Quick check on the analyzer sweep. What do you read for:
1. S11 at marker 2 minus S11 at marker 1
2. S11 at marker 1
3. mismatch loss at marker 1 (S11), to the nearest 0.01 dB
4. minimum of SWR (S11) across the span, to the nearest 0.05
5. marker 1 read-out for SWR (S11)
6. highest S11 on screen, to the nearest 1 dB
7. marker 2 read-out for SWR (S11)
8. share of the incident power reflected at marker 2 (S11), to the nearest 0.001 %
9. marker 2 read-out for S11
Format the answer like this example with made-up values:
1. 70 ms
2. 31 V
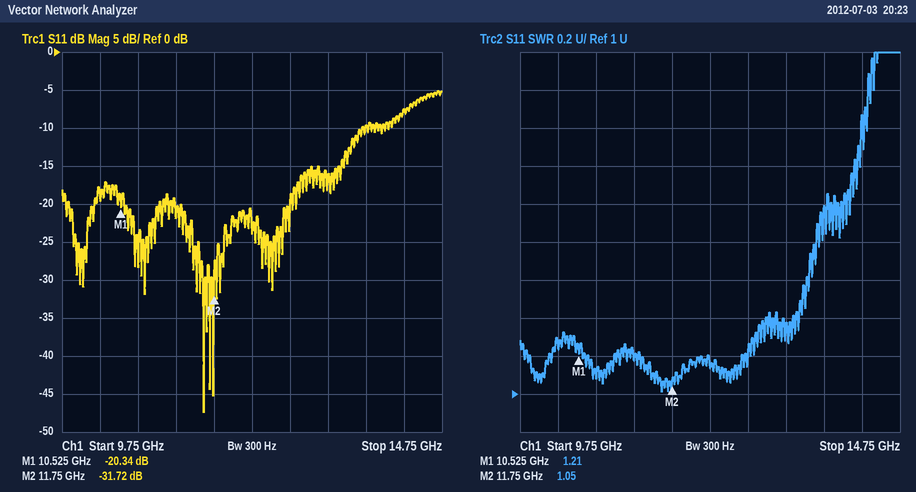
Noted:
1. -11.38 dB
2. -20.34 dB
3. 0.04 dB
4. 1.00
5. 1.21
6. -5 dB
7. 1.05
8. 0.067 %
9. -31.72 dB
